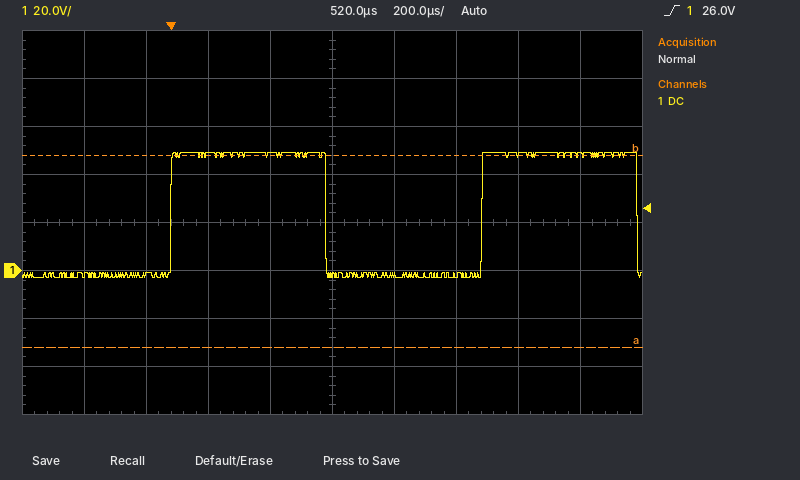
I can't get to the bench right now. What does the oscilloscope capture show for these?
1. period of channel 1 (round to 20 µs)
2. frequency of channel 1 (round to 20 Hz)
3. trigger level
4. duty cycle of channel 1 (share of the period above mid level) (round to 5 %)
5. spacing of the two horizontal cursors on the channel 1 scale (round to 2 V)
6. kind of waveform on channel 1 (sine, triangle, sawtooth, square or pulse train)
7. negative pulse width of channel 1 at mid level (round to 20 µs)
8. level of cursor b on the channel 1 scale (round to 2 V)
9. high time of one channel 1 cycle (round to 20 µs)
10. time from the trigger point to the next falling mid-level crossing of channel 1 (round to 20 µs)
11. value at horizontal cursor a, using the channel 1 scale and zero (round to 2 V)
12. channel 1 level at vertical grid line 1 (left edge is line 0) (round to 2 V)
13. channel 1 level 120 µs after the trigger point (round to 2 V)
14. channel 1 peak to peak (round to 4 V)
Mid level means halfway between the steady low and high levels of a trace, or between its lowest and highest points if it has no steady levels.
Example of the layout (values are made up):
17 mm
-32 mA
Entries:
1.00 ms
1.00 kHz
26.0 V
50 %
80 V
square
500 µs
48 V
500 µs
500 µs
-32 V
-2 V
48 V
52 V
